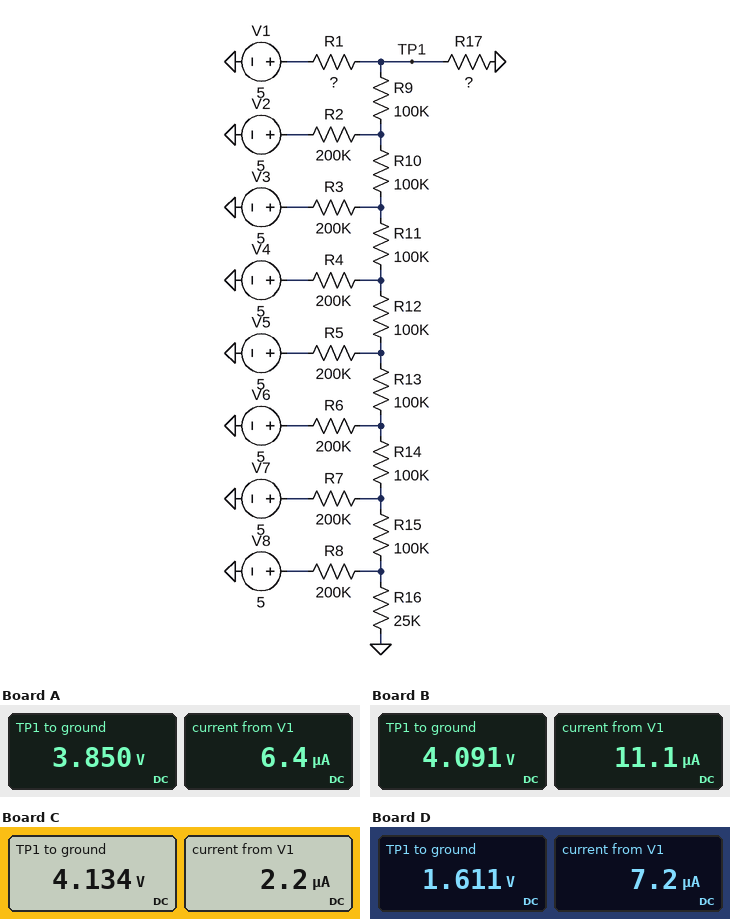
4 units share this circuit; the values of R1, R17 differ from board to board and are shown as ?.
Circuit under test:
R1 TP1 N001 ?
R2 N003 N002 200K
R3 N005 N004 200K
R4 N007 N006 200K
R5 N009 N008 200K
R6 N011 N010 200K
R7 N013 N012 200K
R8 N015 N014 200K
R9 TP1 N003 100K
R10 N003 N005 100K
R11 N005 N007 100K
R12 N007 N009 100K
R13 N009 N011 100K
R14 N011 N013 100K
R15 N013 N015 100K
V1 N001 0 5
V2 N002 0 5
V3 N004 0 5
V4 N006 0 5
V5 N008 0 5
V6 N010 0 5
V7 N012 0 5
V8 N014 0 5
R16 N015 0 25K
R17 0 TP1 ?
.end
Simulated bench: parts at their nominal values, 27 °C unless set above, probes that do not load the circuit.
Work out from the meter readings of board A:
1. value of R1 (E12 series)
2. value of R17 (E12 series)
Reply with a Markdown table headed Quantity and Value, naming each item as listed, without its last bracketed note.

| Quantity | Value |
|---|---|
| value of R1 | 180 kΩ |
| value of R17 | 330 kΩ |
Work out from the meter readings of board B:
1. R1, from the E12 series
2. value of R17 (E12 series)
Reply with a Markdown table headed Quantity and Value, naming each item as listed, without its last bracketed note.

| Quantity | Value |
|---|---|
| R1, from the E12 series | 82 kΩ |
| value of R17 | 270 kΩ |
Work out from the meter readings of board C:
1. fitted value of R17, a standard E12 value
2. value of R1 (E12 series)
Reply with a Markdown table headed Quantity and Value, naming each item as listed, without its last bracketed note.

| Quantity | Value |
|---|---|
| fitted value of R17, a standard E12 value | 680 kΩ |
| value of R1 | 390 kΩ |
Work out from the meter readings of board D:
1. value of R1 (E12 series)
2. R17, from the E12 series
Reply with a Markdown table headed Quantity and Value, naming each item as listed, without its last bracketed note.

| Quantity | Value |
|---|---|
| value of R1 | 470 kΩ |
| R17, from the E12 series | 68 kΩ |
